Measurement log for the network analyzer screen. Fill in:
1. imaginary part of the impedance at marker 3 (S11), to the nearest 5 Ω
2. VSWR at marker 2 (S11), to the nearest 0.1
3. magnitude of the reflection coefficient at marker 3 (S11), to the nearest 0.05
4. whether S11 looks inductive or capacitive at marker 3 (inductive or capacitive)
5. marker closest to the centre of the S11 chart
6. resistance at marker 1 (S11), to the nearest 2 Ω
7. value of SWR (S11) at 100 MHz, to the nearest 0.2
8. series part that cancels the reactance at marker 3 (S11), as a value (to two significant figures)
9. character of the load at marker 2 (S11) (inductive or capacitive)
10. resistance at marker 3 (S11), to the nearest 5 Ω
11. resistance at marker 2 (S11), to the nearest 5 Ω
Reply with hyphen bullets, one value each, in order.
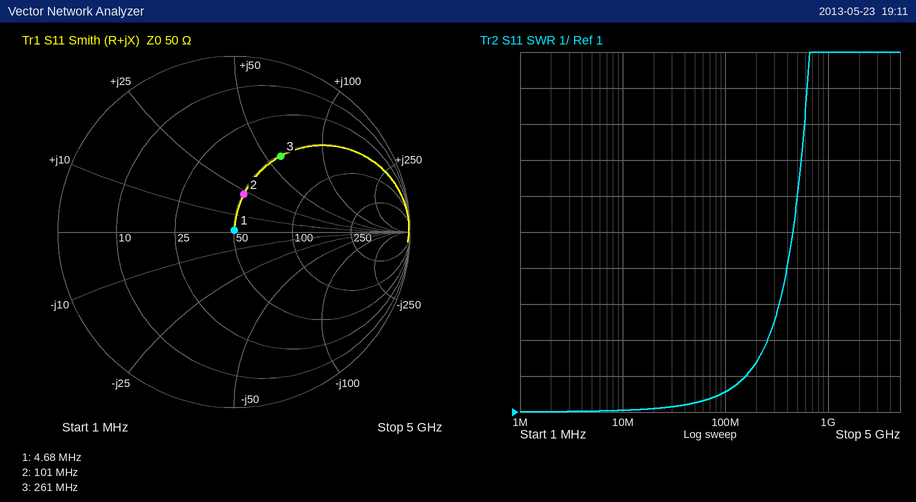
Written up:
- +60 Ω
- 1.6
- 0.50
- inductive
- marker 1
- 50 Ω
- 1.6
- 10 pF
- inductive
- 50 Ω
- 50 Ω
